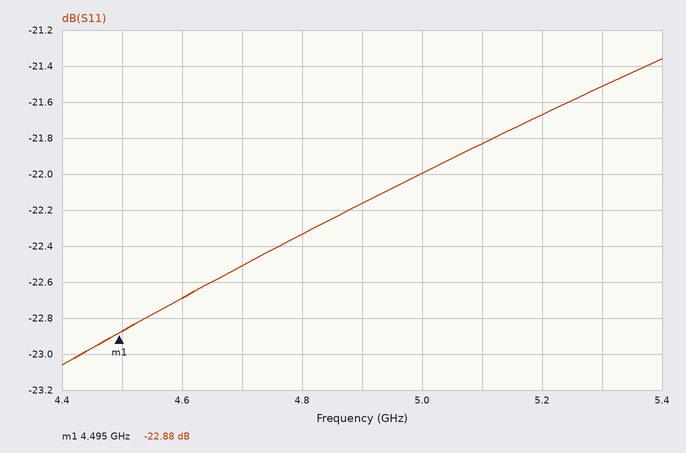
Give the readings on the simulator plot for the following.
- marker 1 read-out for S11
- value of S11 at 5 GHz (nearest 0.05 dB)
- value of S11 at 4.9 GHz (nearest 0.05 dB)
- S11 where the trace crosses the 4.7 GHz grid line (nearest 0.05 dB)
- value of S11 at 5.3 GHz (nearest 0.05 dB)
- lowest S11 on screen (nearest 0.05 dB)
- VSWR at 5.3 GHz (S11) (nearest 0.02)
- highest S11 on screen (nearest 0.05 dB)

-22.88 dB
-22.00 dB
-22.15 dB
-22.50 dB
-21.50 dB
-23.05 dB
1.18
-21.35 dB
